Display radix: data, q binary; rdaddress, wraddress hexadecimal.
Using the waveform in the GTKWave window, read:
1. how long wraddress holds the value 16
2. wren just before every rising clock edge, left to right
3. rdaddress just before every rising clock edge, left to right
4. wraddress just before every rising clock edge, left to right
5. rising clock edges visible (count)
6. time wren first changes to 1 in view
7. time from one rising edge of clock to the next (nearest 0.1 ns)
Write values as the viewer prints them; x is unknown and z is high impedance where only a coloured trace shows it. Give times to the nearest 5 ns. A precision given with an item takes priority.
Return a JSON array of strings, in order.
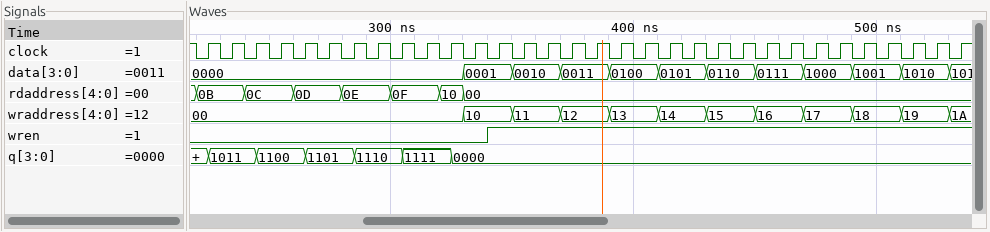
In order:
["20 ns", "0 0 0 0 0 0 0 0 0 0 0 0 1 1 1 1 1 1 1 1 1 1 1 1 1 1 1 1 1 1 1 1", "0B, 0B, 0C, 0C, 0D, 0D, 0E, 0E, 0F, 0F, 10, 00, 00, 00, 00, 00, 00, 00, 00, 00, 00, 00, 00, 00, 00, 00, 00, 00, 00, 00, 00, 00", "00, 00, 00, 00, 00, 00, 00, 00, 00, 00, 00, 10, 10, 11, 11, 12, 12, 13, 13, 14, 14, 15, 15, 16, 16, 17, 17, 18, 18, 19, 19, 1A", "32", "340 ns", "10 ns"]
